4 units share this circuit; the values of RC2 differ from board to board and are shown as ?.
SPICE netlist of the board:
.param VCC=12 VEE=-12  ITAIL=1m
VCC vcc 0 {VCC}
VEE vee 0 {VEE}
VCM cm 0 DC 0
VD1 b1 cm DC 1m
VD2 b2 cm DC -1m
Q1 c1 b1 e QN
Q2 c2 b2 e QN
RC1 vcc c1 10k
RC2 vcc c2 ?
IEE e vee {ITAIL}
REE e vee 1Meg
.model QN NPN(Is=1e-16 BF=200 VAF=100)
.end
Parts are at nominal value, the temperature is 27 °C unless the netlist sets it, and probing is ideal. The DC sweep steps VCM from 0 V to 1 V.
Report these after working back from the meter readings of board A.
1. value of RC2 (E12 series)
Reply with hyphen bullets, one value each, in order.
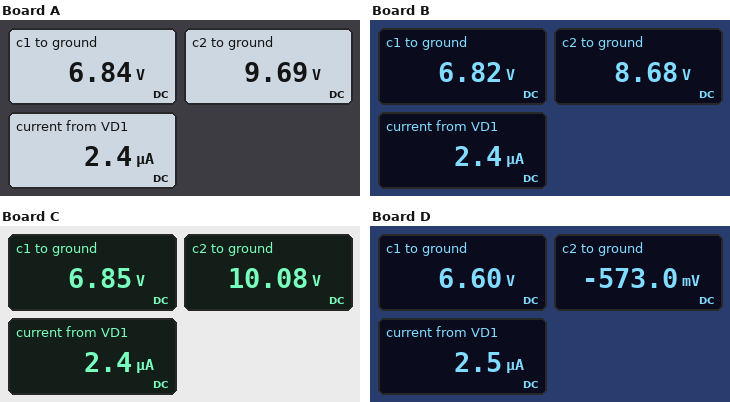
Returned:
- 4.7 kΩ
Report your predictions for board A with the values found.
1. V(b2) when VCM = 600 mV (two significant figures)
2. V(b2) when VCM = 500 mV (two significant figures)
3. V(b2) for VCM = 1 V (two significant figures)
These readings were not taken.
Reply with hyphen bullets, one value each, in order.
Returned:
- 600 mV
- 500 mV
- 1.0 V
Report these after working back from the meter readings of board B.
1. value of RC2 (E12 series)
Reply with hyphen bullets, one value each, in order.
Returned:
- 6.8 kΩ
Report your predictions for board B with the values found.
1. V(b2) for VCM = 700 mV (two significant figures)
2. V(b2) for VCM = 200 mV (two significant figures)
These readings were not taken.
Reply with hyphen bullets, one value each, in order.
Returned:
- 700 mV
- 200 mV
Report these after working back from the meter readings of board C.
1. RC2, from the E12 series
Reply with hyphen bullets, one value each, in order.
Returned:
- 3.9 kΩ
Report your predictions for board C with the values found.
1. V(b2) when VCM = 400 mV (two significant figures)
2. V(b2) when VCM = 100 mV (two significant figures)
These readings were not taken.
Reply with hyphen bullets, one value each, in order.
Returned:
- 400 mV
- 99 mV
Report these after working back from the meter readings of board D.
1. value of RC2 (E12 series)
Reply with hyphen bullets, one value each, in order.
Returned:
- 27 kΩ
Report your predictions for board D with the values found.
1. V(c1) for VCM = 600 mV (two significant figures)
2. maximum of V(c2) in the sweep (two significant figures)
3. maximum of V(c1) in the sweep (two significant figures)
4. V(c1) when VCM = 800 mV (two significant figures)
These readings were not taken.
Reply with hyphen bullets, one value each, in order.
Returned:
- 6.5 V
- 320 mV
- 6.6 V
- 6.5 V
